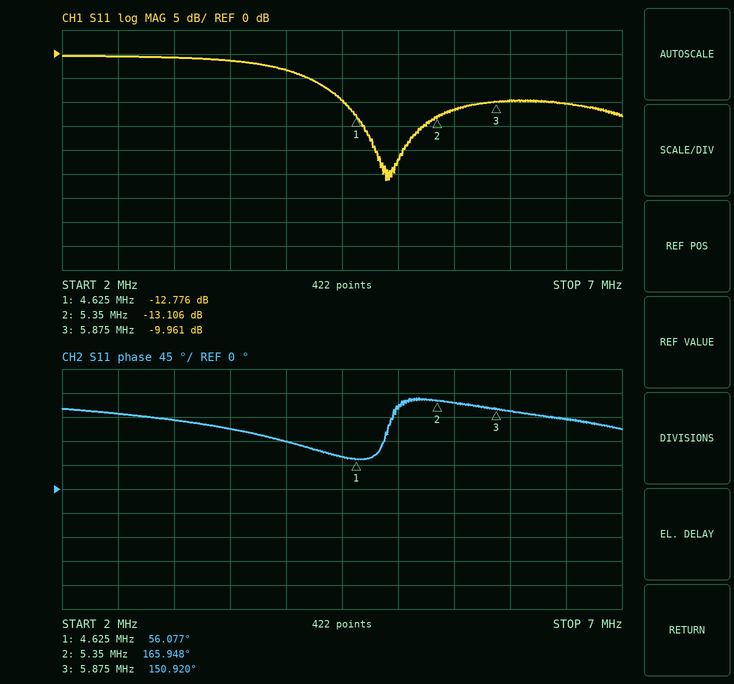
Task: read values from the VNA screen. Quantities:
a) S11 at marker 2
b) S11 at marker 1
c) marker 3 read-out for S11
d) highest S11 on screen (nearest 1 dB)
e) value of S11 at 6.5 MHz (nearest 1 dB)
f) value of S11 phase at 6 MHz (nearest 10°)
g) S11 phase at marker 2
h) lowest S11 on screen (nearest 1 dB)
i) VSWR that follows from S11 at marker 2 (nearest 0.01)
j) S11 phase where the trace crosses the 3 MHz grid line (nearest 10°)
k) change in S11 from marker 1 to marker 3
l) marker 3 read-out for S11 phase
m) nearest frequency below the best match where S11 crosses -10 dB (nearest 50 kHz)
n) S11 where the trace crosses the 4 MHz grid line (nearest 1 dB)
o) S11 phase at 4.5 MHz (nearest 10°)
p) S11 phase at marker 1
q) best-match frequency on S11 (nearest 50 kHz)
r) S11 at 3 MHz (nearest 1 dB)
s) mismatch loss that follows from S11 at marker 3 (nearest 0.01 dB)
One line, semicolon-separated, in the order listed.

-13.106 dB; -12.776 dB; -9.961 dB; 0 dB; -10 dB; 150°; 165.948°; -26 dB; 1.57; 130°; 2.815 dB; 150.920°; 4.50 MHz; -3 dB; 60°; 56.077°; 4.90 MHz; -1 dB; 0.46 dB
